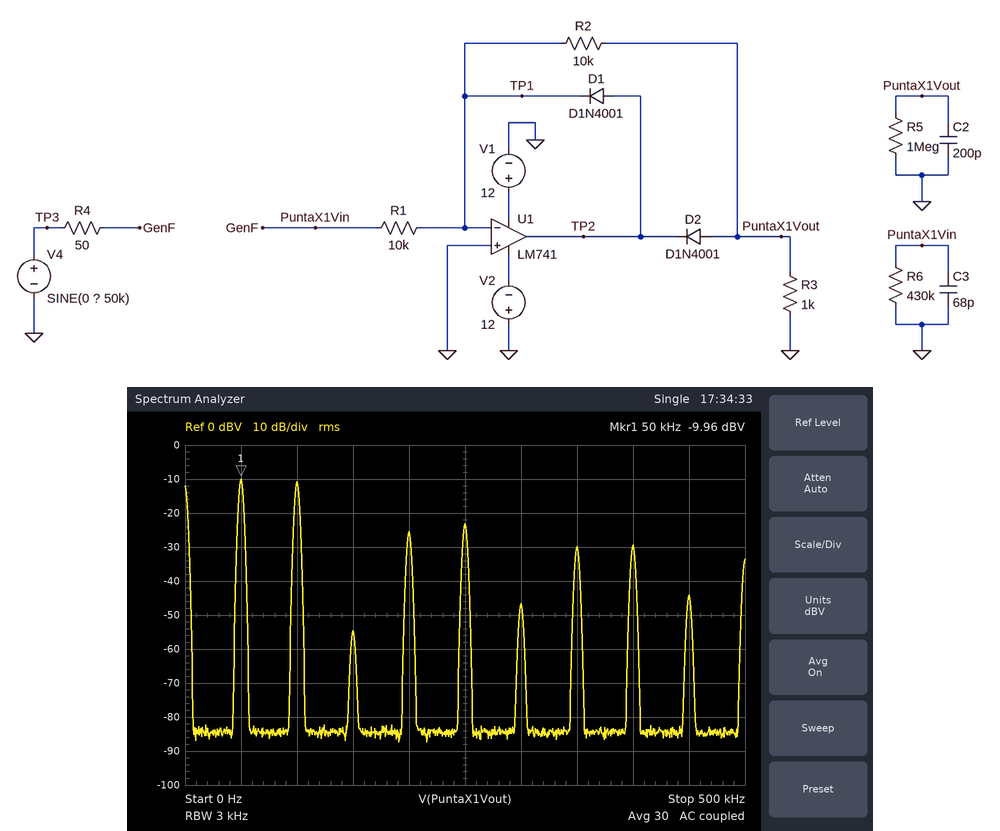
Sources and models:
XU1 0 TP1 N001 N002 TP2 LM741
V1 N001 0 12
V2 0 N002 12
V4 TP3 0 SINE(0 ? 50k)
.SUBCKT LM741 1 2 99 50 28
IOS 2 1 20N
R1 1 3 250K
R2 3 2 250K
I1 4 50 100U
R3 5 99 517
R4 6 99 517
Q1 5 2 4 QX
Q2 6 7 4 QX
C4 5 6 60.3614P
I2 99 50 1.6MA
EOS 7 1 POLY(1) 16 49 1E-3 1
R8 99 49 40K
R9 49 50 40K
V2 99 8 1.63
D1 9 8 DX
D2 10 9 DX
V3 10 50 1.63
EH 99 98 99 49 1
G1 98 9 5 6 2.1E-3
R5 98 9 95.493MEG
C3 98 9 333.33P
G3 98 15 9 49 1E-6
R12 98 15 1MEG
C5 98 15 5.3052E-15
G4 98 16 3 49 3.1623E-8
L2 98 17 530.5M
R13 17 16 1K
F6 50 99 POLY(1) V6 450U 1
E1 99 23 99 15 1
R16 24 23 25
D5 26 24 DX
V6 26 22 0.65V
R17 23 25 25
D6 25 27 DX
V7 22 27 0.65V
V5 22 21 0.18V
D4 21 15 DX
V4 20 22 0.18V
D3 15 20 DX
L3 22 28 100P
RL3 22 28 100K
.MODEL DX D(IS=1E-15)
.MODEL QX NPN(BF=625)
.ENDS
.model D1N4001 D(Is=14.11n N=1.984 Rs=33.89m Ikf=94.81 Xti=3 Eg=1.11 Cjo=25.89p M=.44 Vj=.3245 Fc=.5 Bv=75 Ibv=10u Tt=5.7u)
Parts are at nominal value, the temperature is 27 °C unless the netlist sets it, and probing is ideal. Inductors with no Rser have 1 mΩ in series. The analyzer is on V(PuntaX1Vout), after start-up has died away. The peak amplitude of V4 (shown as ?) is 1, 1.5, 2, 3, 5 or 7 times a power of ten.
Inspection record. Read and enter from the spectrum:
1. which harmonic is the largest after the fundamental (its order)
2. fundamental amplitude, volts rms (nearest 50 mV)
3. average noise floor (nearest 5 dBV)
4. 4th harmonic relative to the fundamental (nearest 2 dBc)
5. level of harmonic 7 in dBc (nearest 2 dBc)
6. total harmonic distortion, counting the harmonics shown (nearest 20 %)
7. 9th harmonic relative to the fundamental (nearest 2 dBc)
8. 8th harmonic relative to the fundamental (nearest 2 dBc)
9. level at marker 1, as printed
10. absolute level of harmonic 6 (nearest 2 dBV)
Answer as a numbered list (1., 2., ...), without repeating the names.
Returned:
1. 2
2. 300 mV
3. -85 dBV
4. -16 dBc
5. -20 dBc
6. 100 %
7. -34 dBc
8. -20 dBc
9. -9.96 dBV
10. -46 dBV
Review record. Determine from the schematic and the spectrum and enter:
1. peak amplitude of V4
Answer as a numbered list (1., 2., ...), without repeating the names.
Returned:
1. 10 V
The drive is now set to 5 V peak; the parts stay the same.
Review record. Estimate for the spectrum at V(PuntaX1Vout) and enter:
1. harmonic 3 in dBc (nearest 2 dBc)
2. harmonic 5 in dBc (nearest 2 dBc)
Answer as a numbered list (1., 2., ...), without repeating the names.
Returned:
1. -16 dBc
2. -14 dBc
